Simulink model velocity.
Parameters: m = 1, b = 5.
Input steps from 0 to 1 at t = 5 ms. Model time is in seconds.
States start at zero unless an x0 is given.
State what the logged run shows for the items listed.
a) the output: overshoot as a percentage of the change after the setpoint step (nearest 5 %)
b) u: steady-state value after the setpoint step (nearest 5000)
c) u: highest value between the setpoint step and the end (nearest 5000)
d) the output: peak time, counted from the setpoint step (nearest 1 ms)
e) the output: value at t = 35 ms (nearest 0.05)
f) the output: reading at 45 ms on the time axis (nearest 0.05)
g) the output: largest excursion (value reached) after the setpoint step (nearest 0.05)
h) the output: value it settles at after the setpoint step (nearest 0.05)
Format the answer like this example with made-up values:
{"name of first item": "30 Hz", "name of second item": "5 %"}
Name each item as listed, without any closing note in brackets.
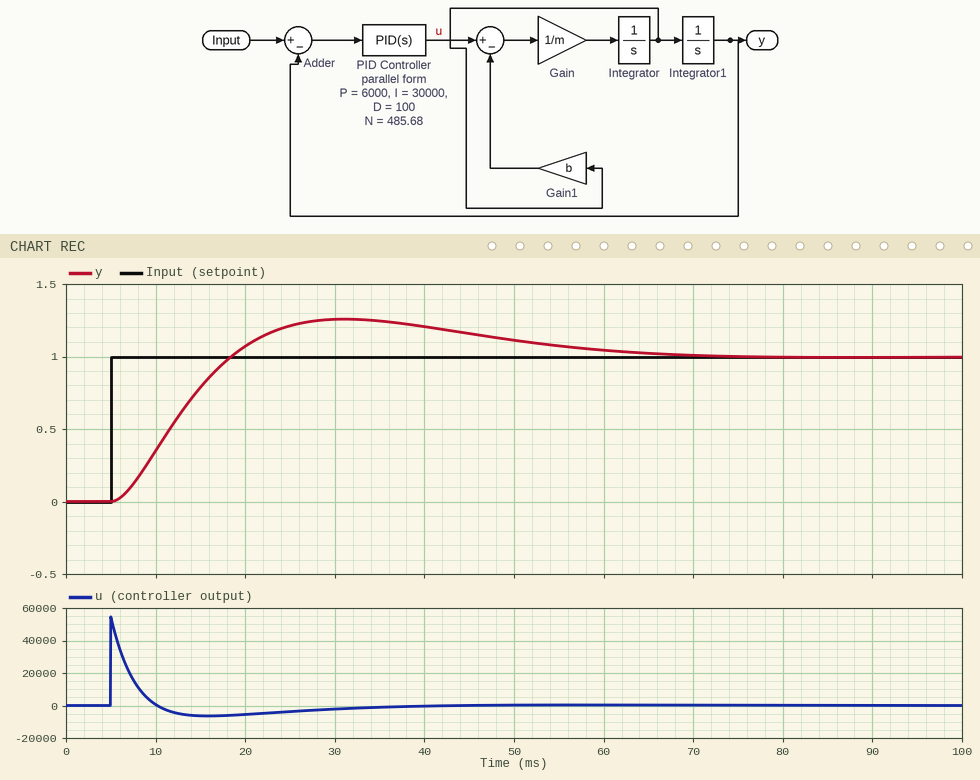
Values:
{"the output: overshoot as a percentage of the change after the setpoint step": "25 %", "u: steady-state value after the setpoint step": "0", "u: highest value between the setpoint step and the end": "55000", "the output: peak time, counted from the setpoint step": "26 ms", "the output: value at t = 35 ms": "1.25", "the output: reading at 45 ms on the time axis": "1.15", "the output: largest excursion (value reached) after the setpoint step": "1.25", "the output: value it settles at after the setpoint step": "1.00"}
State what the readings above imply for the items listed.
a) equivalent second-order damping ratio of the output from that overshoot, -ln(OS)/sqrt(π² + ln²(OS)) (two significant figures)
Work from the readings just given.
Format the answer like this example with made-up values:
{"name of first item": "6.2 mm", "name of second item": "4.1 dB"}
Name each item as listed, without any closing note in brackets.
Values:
{"equivalent second-order damping ratio of the output from that overshoot, -ln(OS)/sqrt(π² + ln²(OS))": "0.40"}
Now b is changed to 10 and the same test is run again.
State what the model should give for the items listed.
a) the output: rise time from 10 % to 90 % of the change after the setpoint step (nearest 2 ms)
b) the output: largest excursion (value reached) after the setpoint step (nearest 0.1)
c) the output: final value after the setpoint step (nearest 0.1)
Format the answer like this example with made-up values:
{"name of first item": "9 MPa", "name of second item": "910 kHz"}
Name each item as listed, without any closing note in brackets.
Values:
{"the output: rise time from 10 % to 90 % of the change after the setpoint step": "10 ms", "the output: largest excursion (value reached) after the setpoint step": "1.2", "the output: final value after the setpoint step": "1.0"}
